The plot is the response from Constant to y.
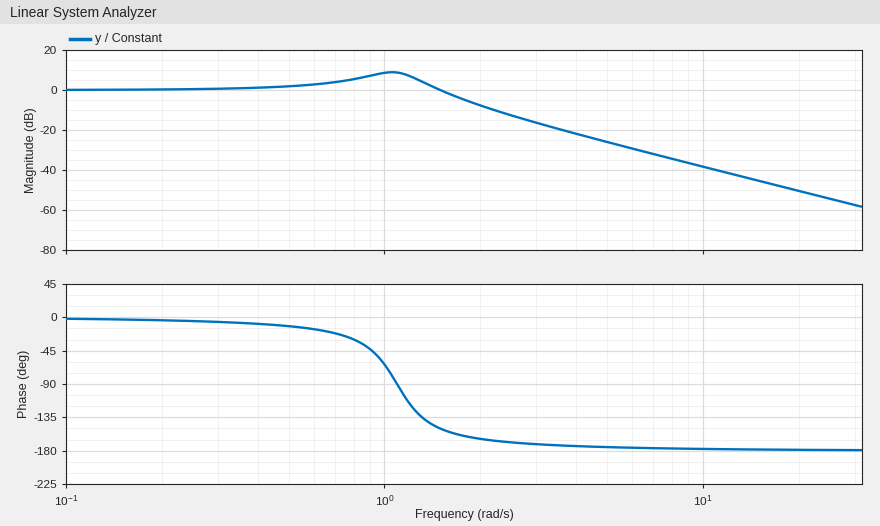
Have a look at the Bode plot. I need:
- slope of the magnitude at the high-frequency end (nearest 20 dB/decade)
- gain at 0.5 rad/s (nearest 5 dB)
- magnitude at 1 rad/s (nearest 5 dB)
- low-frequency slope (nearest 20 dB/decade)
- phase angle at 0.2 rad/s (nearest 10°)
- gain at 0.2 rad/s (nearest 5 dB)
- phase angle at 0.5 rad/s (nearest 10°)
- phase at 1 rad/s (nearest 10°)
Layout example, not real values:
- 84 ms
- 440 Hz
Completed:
- -40 dB/decade
- 0 dB
- 10 dB
- 0 dB/decade
- 0°
- 0 dB
- -10°
- -60°
